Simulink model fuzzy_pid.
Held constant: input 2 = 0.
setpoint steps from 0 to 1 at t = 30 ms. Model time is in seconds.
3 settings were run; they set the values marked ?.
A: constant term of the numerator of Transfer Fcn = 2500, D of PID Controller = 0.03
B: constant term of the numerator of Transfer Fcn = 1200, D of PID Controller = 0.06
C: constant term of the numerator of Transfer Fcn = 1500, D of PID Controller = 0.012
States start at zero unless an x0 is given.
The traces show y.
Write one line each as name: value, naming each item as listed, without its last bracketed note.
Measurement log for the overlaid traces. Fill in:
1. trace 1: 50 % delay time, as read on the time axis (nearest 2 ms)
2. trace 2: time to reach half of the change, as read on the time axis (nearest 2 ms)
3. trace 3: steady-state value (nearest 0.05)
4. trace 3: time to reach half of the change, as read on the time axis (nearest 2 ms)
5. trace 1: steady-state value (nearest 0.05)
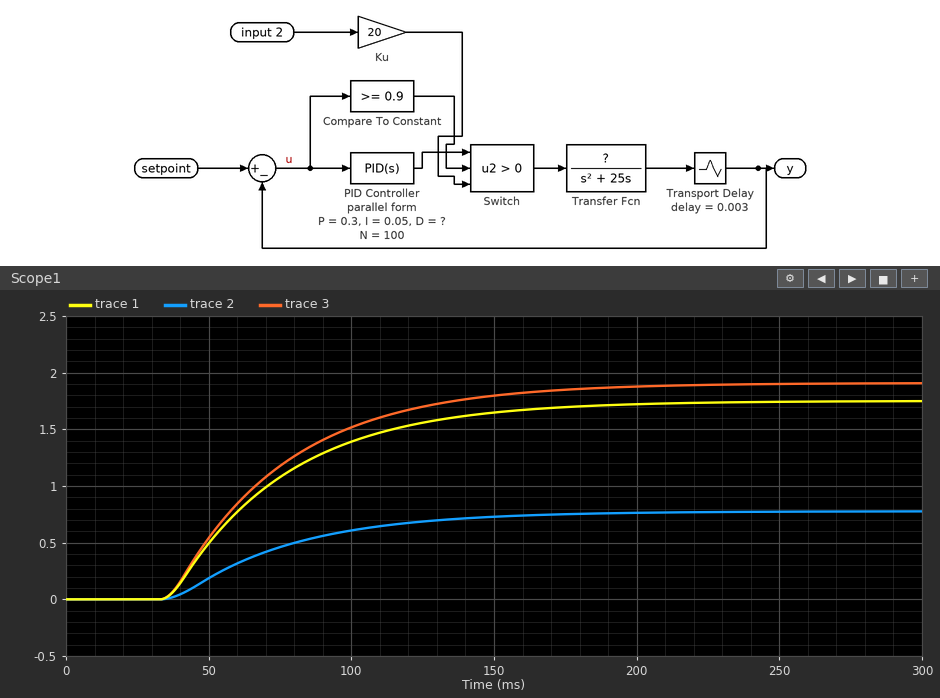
trace 1: 50 % delay time, as read on the time axis: 64 ms
trace 2: time to reach half of the change, as read on the time axis: 66 ms
trace 3: steady-state value: 1.90
trace 3: time to reach half of the change, as read on the time axis: 64 ms
trace 1: steady-state value: 1.75
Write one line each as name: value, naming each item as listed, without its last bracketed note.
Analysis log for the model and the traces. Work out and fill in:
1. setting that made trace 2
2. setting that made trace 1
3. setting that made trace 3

setting that made trace 2: C
setting that made trace 1: B
setting that made trace 3: A
